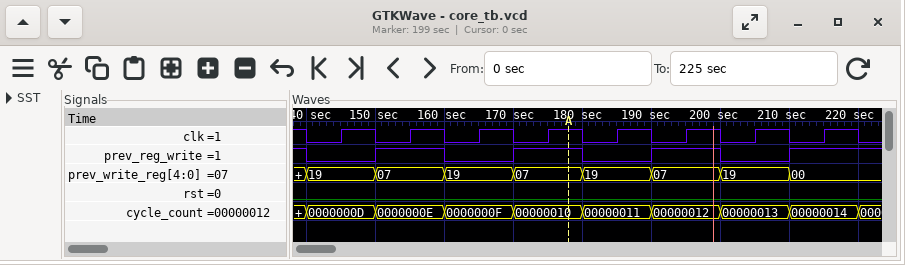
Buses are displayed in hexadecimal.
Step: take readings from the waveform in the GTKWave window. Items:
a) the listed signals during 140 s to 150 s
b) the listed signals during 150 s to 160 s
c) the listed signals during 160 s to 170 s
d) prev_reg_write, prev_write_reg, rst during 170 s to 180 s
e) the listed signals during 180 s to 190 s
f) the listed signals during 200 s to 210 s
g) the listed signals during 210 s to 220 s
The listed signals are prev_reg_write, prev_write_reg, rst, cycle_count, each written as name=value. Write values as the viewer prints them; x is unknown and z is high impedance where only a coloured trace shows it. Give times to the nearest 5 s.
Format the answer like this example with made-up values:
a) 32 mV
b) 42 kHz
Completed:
a) prev_reg_write=0, prev_write_reg=19, rst=0, cycle_count=0000000D
b) prev_reg_write=1, prev_write_reg=07, rst=0, cycle_count=0000000E
c) prev_reg_write=0, prev_write_reg=19, rst=0, cycle_count=0000000F
d) prev_reg_write=1, prev_write_reg=07, rst=0
e) prev_reg_write=0, prev_write_reg=19, rst=0, cycle_count=00000011
f) prev_reg_write=0, prev_write_reg=19, rst=0, cycle_count=00000013
g) prev_reg_write=1, prev_write_reg=00, rst=0, cycle_count=00000014
